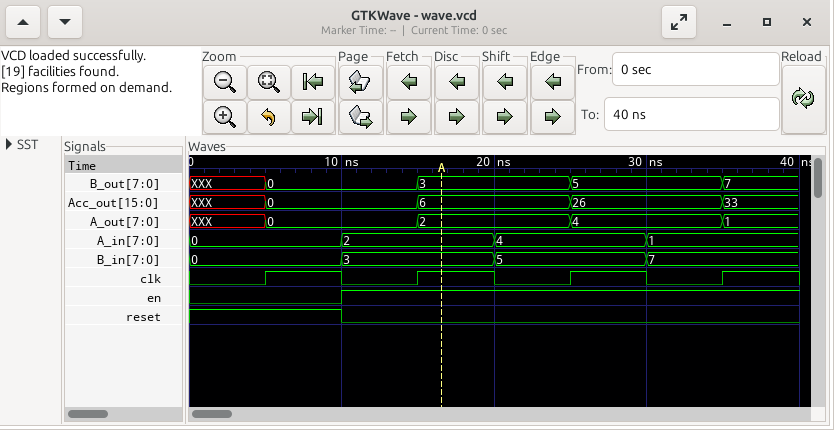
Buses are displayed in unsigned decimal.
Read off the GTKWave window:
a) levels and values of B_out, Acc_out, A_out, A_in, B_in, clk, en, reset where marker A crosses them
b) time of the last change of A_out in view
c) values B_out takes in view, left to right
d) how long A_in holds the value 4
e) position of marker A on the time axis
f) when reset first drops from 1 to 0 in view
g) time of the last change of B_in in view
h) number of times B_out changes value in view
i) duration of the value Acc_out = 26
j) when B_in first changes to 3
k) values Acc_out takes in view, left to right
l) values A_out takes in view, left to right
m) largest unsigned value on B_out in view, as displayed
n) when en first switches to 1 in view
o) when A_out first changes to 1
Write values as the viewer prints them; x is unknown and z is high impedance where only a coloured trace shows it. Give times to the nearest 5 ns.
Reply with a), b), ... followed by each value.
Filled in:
a) B_out=3, Acc_out=6, A_out=2, A_in=2, B_in=3, clk=1, en=1, reset=0
b) 35 ns
c) XXX, 0, 3, 5, 7
d) 10 ns
e) 15 ns
f) 10 ns
g) 30 ns
h) 4
i) 10 ns
j) 10 ns
k) XXX, 0, 6, 26, 33
l) XXX, 0, 2, 4, 1
m) 7
n) 10 ns
o) 35 ns
